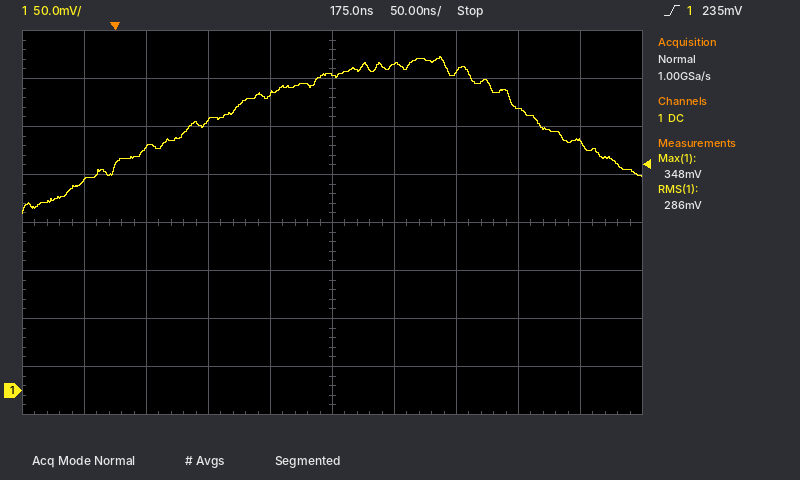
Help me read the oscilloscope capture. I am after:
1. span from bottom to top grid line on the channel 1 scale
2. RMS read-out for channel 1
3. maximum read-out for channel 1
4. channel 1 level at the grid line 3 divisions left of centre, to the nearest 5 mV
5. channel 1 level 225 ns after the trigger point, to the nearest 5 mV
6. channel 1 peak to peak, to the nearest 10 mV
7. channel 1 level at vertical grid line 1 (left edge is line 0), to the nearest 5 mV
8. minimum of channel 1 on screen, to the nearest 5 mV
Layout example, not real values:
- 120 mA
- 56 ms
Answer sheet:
- 400 mV
- 286 mV
- 348 mV
- 255 mV
- 340 mV
- 160 mV
- 220 mV
- 185 mV
